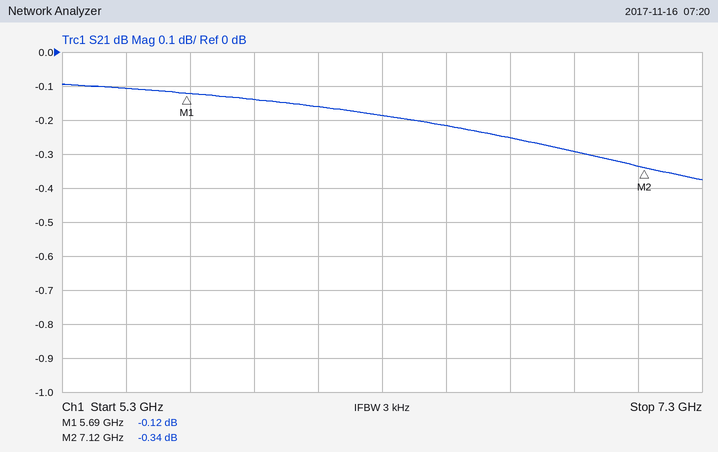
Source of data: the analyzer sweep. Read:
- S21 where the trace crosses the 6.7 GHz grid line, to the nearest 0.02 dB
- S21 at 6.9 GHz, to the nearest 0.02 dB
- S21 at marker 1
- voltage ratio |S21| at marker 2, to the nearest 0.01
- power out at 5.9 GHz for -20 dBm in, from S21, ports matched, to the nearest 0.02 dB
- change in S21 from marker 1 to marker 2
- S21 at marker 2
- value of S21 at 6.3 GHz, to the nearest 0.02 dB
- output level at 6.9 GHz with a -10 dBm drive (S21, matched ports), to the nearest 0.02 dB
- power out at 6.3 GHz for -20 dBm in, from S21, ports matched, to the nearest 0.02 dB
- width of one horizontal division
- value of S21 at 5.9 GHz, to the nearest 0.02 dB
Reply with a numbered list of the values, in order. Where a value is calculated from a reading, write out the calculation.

1. -0.26 dB
2. -0.30 dB
3. -0.12 dB
4. 10^(-0.34/20) ≈ 0.96
5. -20 dBm + (-0.14 dB) = -20.14 dBm
6. -0.34 − (-0.12) = -0.22 dB
7. -0.34 dB
8. -0.18 dB
9. -10 dBm + (-0.30 dB) = -10.30 dBm
10. -20 dBm + (-0.18 dB) = -20.18 dBm
11. 200 MHz
12. -0.14 dB
